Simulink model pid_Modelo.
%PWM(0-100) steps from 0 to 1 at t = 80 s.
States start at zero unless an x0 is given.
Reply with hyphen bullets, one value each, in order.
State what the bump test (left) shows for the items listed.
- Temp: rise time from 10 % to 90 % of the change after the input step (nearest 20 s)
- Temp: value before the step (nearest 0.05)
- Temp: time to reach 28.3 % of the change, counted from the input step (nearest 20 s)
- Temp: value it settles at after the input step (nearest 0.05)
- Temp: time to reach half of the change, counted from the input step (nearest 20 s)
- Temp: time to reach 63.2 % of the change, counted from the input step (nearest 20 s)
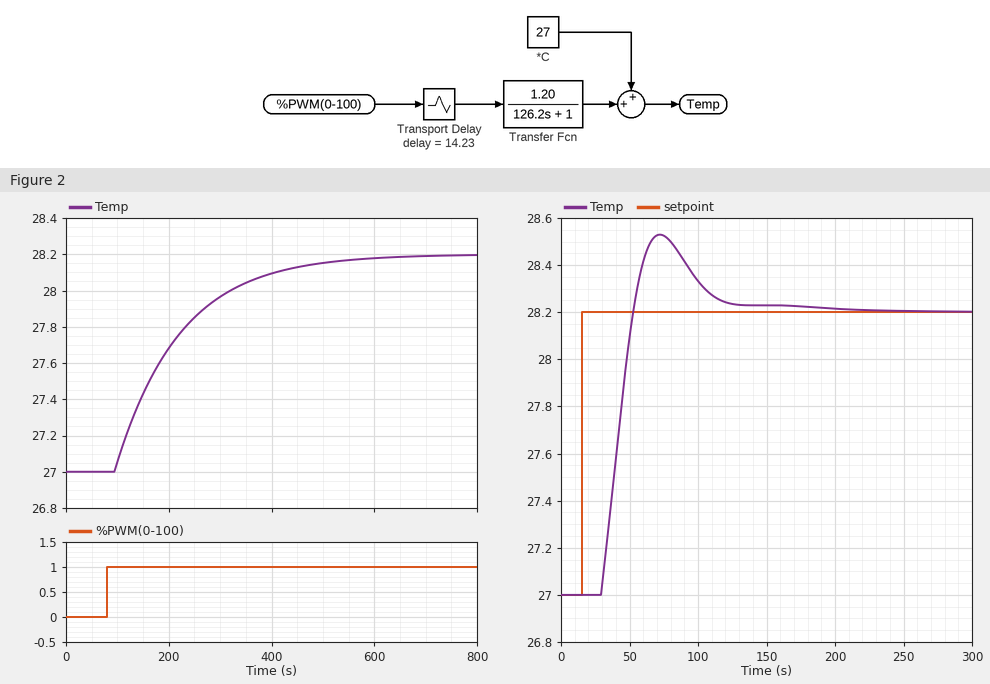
- 280 s
- 27.00
- 60 s
- 28.20
- 100 s
- 140 s
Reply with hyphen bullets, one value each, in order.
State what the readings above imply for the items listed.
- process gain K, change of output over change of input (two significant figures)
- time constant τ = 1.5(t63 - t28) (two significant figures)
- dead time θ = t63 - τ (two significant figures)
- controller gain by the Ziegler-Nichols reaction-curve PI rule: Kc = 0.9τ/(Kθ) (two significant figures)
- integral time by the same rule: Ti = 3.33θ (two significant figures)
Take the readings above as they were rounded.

- 1.2
- 120 s
- 20 s
- 4.5
- 67 s
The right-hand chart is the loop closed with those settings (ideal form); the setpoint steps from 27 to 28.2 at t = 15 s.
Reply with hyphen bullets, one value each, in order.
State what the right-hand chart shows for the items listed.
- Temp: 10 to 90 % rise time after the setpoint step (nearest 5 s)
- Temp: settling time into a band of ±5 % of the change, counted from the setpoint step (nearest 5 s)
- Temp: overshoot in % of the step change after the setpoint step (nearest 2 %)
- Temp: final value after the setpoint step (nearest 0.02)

- 20 s
- 100 s
- 28 %
- 28.20
